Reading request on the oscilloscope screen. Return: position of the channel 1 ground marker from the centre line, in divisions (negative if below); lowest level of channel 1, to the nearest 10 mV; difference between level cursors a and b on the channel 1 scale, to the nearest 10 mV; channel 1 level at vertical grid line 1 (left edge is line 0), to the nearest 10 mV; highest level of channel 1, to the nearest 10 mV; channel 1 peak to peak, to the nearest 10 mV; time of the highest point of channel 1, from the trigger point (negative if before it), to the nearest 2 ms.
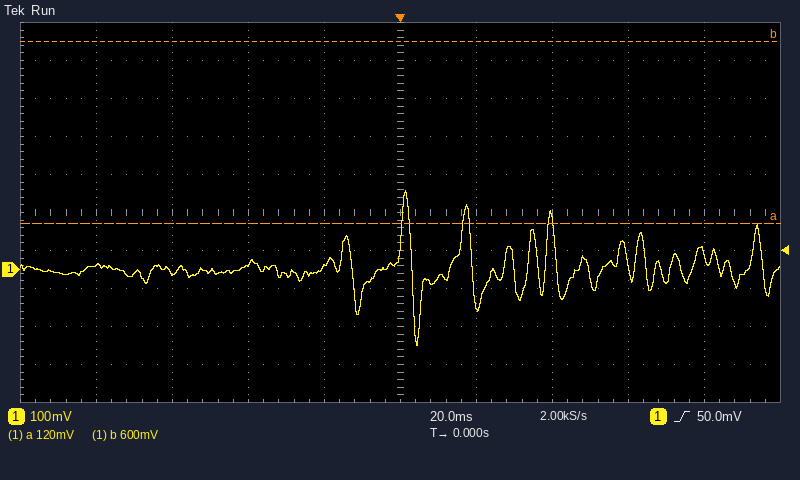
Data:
-1.5 div
-200 mV
480 mV
10 mV
210 mV
410 mV
+2 ms
